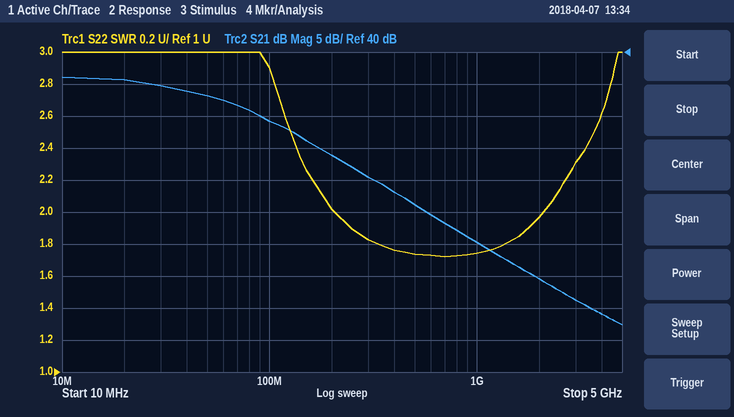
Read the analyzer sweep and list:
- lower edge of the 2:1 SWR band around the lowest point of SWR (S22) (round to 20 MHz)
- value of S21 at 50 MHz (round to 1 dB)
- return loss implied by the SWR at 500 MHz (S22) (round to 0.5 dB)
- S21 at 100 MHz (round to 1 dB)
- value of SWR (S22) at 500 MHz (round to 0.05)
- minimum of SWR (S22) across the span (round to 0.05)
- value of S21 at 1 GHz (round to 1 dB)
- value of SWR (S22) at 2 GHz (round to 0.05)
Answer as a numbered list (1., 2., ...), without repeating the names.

1. 200 MHz
2. 33 dB
3. 11.5 dB
4. 29 dB
5. 1.75
6. 1.70
7. 10 dB
8. 1.95
